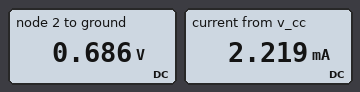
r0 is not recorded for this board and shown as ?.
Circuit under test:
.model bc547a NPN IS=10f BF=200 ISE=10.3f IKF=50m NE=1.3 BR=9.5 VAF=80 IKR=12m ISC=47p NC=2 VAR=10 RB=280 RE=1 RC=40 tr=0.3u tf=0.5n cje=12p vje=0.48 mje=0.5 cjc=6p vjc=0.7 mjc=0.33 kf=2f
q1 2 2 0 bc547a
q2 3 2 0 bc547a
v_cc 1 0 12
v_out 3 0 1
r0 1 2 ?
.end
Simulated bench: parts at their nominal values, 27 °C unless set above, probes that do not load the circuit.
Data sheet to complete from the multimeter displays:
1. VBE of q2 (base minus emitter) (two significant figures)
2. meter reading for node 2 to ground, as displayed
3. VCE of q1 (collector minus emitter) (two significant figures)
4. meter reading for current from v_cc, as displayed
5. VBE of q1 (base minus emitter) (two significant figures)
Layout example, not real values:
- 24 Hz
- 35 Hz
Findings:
- 690 mV
- 0.686 V
- 690 mV
- 2.219 mA
- 690 mV
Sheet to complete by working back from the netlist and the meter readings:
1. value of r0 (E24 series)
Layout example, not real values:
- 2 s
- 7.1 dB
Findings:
- 5.1 kΩ
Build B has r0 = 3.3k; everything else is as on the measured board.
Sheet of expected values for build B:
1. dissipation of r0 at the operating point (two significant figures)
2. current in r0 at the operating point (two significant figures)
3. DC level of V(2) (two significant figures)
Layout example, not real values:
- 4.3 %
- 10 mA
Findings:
- 39 mW
- 3.4 mA
- 700 mV
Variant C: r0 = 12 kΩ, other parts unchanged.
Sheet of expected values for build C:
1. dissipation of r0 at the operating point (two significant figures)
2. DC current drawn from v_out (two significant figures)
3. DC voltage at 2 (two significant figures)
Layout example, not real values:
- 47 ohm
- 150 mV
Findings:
- 11 mW
- 930 µA
- 660 mV
